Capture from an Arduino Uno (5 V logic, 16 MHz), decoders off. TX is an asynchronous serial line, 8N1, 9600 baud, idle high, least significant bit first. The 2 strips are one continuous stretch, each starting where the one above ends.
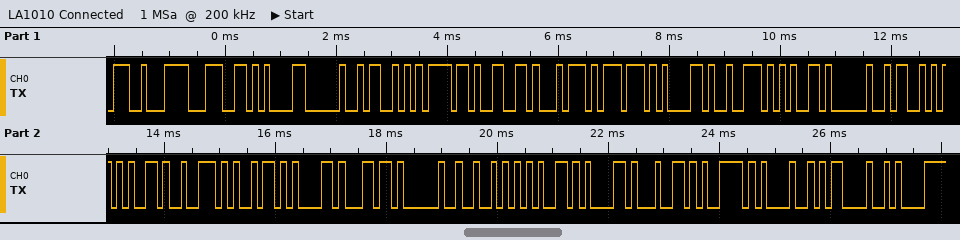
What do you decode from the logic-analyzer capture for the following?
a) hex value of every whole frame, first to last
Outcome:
0xE2 0x9C 0x85 0x20 0x53 0x6F 0x66 0x74 0x77 0x61 0x72 0x65 0x20 0x53 0x65 0x72 0x69 0x61 0x6C 0x20 0x52 0x65 0x61 0x64 0x79 0x21 0x0D 0x0A
